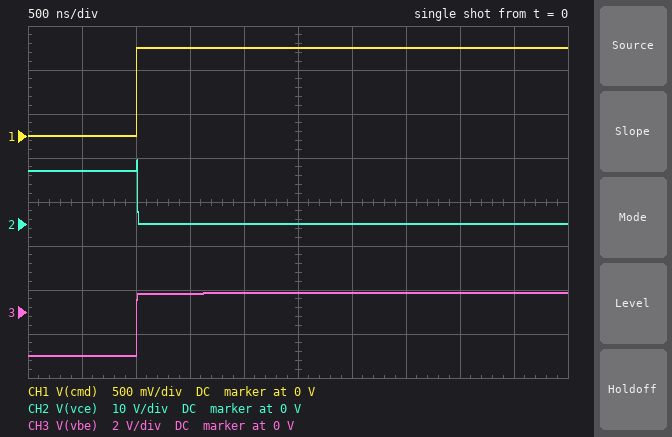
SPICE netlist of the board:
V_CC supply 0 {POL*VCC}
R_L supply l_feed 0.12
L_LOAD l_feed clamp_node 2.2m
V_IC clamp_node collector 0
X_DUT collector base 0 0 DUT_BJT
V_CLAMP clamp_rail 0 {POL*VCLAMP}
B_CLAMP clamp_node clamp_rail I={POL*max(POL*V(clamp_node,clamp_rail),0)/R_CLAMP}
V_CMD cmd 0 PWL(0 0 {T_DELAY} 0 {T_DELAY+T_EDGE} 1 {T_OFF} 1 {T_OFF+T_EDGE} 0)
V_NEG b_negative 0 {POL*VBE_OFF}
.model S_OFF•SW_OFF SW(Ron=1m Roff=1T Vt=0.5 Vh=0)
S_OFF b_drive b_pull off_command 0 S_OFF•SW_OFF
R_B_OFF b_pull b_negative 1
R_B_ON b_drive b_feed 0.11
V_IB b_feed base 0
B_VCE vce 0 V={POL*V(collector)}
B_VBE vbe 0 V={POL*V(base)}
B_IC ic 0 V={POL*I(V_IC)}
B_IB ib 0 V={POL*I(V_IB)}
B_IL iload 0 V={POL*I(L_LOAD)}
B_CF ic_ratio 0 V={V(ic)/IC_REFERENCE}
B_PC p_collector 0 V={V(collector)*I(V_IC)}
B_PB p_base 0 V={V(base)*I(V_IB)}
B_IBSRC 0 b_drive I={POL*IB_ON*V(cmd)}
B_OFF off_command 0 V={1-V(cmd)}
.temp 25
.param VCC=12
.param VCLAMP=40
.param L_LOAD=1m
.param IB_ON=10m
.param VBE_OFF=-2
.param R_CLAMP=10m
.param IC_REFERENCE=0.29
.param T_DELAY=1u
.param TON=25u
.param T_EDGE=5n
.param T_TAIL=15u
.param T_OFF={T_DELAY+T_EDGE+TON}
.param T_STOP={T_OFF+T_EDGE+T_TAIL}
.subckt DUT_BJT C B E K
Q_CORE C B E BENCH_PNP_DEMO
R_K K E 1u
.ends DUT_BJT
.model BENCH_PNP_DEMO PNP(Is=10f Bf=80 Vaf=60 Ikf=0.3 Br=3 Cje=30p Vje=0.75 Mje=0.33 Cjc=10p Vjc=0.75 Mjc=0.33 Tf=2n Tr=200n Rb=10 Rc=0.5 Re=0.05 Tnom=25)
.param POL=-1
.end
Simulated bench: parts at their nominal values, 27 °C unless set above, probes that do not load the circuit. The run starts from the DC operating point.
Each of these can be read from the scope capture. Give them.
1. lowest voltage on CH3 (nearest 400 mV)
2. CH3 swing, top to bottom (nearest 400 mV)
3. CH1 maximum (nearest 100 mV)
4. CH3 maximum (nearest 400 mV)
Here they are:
-2.0 V
2.8 V
1.0 V
800 mV
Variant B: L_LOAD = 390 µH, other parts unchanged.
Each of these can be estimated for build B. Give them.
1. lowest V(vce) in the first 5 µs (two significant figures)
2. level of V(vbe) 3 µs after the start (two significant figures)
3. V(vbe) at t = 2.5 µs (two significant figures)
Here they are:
32 mV
880 mV
870 mV
